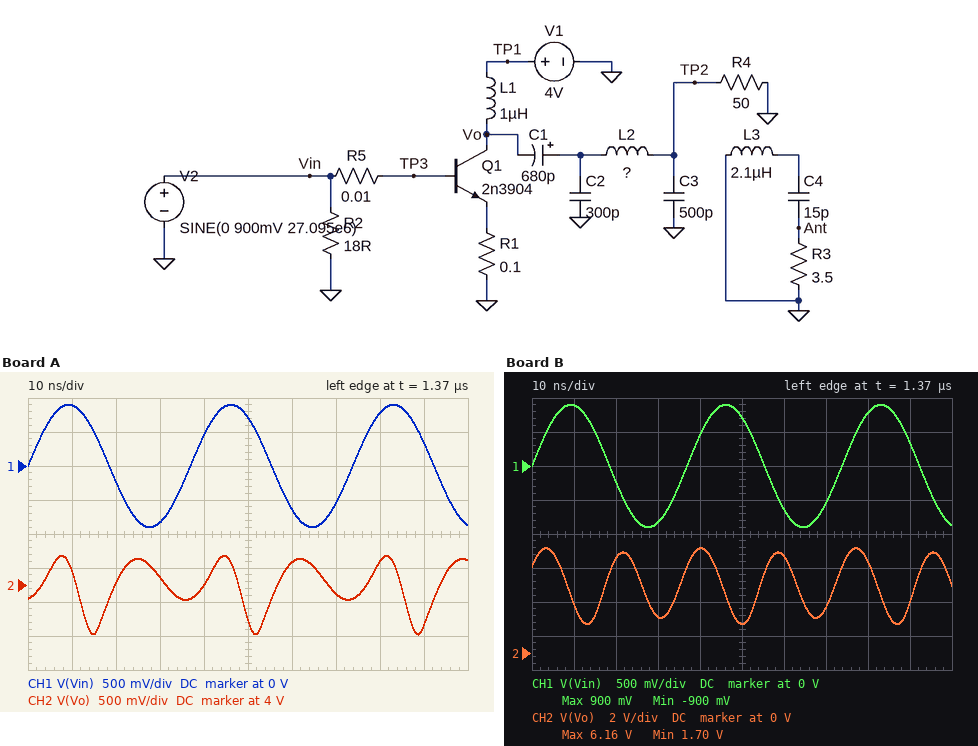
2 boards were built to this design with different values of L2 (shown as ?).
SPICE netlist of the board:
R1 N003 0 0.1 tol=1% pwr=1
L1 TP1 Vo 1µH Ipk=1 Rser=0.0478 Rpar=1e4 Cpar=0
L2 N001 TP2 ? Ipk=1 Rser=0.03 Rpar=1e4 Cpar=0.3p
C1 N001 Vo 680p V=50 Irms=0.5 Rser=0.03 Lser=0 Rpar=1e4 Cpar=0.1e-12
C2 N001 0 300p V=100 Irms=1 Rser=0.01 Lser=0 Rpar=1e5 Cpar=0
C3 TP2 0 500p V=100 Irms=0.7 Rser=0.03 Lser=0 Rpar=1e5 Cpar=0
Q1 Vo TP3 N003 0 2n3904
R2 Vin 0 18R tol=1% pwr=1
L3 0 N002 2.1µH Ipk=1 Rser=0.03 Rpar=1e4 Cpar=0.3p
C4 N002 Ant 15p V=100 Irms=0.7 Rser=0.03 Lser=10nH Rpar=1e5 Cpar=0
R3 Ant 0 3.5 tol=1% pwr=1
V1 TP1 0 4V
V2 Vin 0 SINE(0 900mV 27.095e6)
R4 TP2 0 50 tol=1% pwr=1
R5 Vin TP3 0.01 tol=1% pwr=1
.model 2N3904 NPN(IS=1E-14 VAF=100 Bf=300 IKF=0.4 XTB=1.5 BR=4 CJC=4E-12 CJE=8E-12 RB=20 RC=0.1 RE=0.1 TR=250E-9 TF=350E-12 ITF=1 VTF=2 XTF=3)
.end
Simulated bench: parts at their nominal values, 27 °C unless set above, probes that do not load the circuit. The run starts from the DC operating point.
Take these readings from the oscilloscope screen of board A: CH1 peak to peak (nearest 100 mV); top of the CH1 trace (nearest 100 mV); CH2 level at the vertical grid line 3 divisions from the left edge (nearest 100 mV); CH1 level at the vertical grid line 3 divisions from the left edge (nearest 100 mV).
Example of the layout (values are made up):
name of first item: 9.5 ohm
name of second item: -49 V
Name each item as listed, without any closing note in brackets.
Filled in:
CH1 peak to peak: 1.8 V
top of the CH1 trace: 900 mV
CH2 level at the vertical grid line 3 divisions from the left edge: 4.1 V
CH1 level at the vertical grid line 3 divisions from the left edge: -800 mV
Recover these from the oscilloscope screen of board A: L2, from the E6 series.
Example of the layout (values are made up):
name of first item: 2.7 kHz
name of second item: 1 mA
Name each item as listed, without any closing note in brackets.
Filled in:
L2, from the E6 series: 100 nH
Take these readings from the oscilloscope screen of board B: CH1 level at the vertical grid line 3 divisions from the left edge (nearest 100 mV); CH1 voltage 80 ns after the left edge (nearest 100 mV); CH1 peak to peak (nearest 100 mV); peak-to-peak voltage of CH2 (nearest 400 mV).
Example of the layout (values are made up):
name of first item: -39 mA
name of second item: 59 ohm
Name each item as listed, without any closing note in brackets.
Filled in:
CH1 level at the vertical grid line 3 divisions from the left edge: -800 mV
CH1 voltage 80 ns after the left edge: 800 mV
CH1 peak to peak: 1.8 V
peak-to-peak voltage of CH2: 4.4 V
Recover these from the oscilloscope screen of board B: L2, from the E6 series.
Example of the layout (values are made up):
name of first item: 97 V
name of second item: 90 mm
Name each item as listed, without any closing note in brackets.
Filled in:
L2, from the E6 series: 47 nH
